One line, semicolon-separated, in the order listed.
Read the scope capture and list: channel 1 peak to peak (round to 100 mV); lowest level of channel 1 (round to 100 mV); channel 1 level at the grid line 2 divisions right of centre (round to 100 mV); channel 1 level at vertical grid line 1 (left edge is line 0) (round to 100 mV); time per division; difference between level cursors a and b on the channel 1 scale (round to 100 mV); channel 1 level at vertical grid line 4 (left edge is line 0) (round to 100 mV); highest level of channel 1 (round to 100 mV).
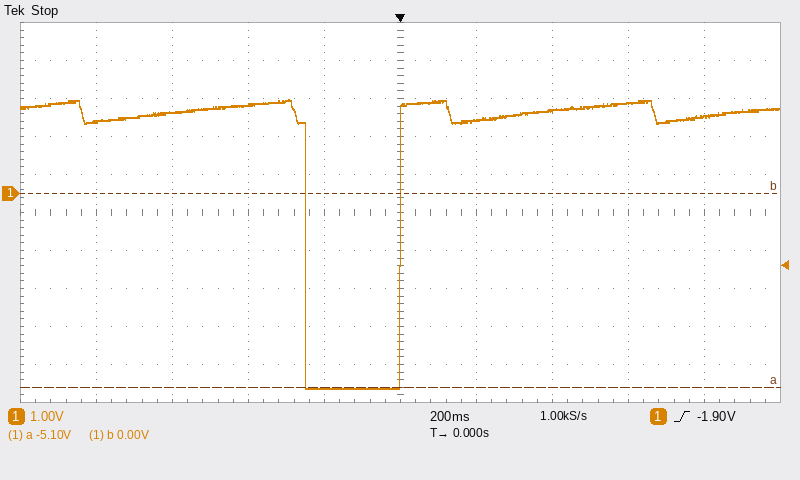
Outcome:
7.6 V; -5.1 V; 2.2 V; 1.9 V; 200 ms; 5.1 V; -5.1 V; 2.5 V
